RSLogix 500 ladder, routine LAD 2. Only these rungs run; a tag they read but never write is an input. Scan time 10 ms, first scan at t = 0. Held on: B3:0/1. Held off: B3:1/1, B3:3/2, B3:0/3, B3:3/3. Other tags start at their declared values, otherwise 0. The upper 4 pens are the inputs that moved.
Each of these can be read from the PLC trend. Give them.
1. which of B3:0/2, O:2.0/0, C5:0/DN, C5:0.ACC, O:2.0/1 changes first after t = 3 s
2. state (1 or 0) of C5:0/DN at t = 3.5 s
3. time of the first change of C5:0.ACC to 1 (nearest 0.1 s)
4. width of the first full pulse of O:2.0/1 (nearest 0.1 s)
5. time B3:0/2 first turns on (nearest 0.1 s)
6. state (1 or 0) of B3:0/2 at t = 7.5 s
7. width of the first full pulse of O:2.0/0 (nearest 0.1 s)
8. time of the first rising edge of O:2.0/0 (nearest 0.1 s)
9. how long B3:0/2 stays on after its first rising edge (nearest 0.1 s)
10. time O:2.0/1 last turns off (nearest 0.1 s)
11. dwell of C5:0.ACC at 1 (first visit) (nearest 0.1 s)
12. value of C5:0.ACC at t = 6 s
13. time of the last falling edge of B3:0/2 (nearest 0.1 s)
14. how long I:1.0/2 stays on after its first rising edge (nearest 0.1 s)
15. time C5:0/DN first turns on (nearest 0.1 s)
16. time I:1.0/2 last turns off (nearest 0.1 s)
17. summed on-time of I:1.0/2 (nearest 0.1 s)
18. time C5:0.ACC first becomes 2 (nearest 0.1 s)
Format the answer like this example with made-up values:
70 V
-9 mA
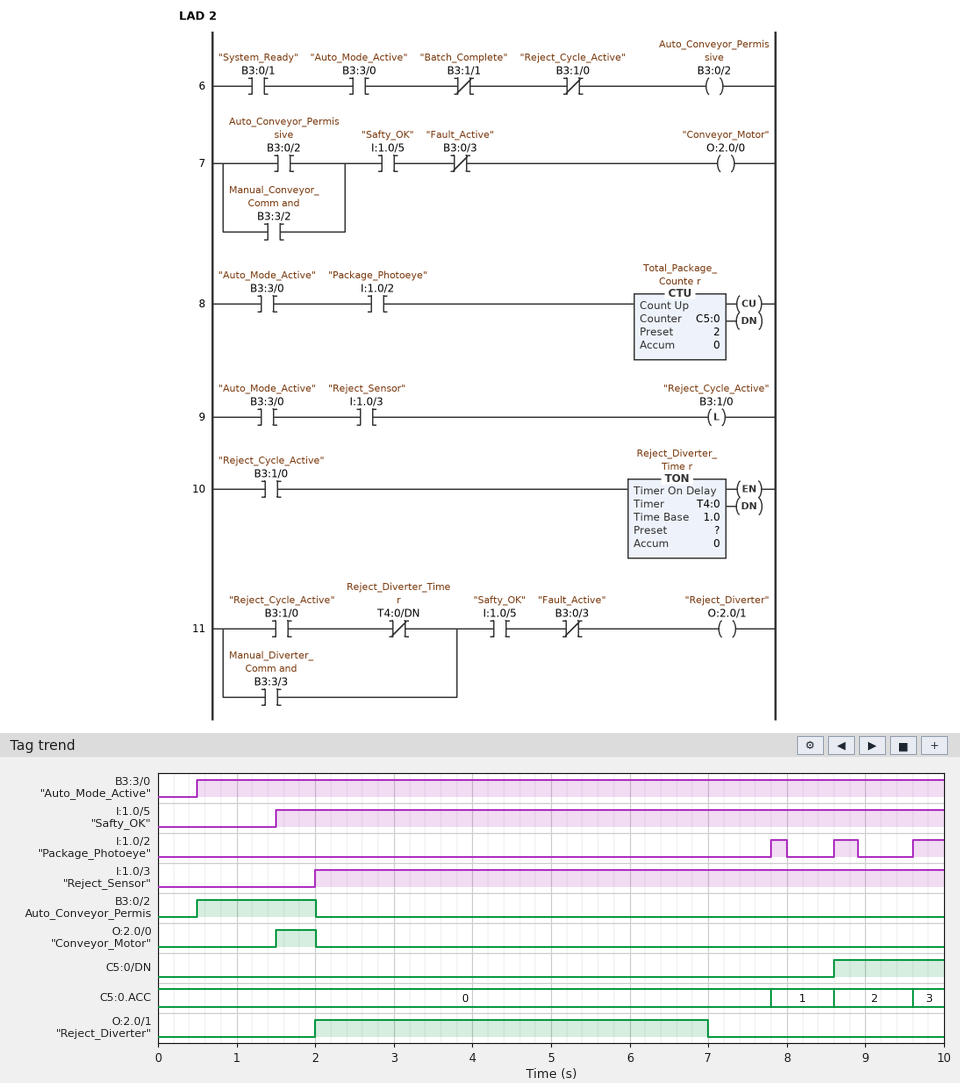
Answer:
O:2.0/1
0
7.8 s
5.0 s
0.5 s
0
0.5 s
1.5 s
1.5 s
7.0 s
0.8 s
0
2.0 s
0.2 s
8.6 s
8.9 s
0.9 s
8.6 s
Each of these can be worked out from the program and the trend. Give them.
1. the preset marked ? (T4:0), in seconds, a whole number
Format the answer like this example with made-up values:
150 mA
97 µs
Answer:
5 s
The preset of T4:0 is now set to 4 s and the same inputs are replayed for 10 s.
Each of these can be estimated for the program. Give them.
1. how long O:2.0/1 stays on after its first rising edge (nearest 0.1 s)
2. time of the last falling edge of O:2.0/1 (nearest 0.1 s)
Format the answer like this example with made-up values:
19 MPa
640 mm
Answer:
4.0 s
6.0 s
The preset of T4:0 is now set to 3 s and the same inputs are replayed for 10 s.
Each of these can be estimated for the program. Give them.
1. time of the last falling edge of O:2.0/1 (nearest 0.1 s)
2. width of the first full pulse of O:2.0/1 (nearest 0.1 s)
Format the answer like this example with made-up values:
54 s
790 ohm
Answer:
5.0 s
3.0 s
